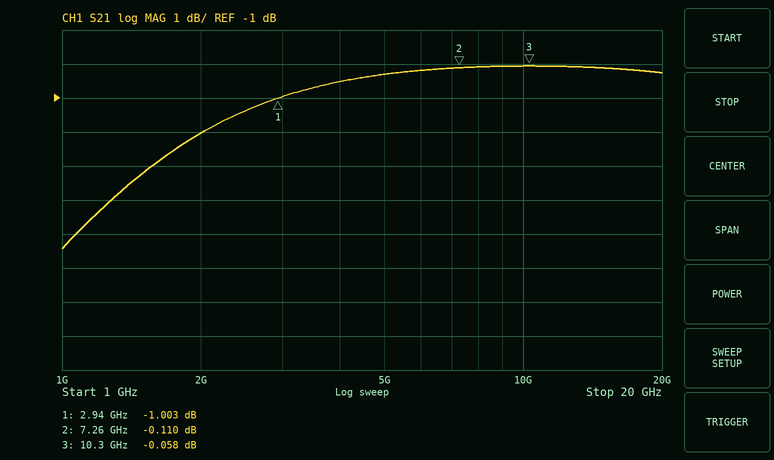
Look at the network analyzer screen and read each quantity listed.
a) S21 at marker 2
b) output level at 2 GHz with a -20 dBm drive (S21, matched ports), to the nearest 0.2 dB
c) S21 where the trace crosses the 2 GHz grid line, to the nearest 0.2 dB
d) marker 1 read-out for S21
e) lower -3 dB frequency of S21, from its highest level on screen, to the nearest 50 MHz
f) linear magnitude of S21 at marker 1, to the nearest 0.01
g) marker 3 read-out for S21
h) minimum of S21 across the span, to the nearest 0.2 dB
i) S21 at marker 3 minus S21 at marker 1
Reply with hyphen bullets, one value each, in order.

- -0.110 dB
- -22.0 dBm
- -2.0 dB
- -1.003 dB
- 1.55 GHz
- 0.89
- -0.058 dB
- -5.4 dB
- 0.945 dB
